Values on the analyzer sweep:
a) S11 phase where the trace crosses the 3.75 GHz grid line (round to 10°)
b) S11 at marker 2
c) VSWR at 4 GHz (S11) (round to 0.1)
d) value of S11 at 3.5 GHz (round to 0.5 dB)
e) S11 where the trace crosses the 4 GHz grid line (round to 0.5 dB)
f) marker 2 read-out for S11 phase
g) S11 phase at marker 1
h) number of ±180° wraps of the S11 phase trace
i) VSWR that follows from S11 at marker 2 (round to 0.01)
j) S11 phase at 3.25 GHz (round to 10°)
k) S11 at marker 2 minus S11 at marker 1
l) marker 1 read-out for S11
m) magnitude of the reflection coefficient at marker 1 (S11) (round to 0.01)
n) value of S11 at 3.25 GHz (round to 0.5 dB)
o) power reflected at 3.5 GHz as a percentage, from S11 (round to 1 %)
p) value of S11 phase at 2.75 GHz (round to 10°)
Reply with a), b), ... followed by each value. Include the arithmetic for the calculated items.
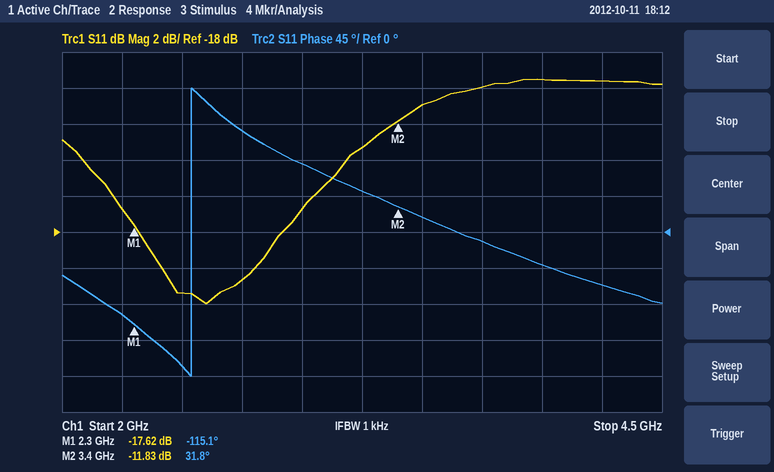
a) -10°
b) -11.83 dB
c) |Γ| = 10^(-9.5/20) = 0.3350; VSWR = (1 + 0.3350)/(1 − 0.3350) ≈ 2.0
d) -11.0 dB
e) -9.5 dB
f) 31.8°
g) -115.1°
h) 1
i) (1 + 0.2562)/(1 − 0.2562) ≈ 1.69
j) 50°
k) -11.83 − (-17.62) = 5.79 dB
l) -17.62 dB
m) 10^(-17.62/20) ≈ 0.13
n) -13.5 dB
o) 10^(-11/10) ≈ 8 %
p) 130°
